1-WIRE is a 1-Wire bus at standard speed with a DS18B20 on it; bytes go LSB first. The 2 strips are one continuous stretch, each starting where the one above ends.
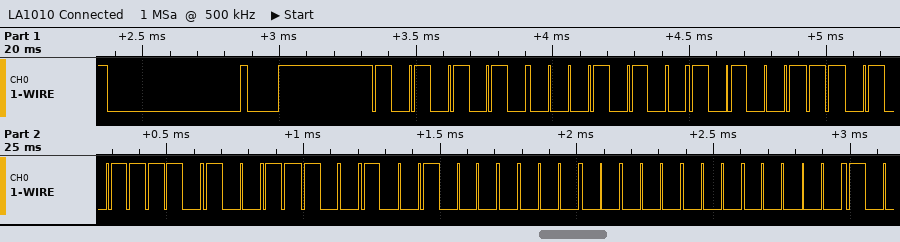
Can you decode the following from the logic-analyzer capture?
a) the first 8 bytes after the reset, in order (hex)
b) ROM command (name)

55 28 E5 7A 39 09 00 00
Match ROM
